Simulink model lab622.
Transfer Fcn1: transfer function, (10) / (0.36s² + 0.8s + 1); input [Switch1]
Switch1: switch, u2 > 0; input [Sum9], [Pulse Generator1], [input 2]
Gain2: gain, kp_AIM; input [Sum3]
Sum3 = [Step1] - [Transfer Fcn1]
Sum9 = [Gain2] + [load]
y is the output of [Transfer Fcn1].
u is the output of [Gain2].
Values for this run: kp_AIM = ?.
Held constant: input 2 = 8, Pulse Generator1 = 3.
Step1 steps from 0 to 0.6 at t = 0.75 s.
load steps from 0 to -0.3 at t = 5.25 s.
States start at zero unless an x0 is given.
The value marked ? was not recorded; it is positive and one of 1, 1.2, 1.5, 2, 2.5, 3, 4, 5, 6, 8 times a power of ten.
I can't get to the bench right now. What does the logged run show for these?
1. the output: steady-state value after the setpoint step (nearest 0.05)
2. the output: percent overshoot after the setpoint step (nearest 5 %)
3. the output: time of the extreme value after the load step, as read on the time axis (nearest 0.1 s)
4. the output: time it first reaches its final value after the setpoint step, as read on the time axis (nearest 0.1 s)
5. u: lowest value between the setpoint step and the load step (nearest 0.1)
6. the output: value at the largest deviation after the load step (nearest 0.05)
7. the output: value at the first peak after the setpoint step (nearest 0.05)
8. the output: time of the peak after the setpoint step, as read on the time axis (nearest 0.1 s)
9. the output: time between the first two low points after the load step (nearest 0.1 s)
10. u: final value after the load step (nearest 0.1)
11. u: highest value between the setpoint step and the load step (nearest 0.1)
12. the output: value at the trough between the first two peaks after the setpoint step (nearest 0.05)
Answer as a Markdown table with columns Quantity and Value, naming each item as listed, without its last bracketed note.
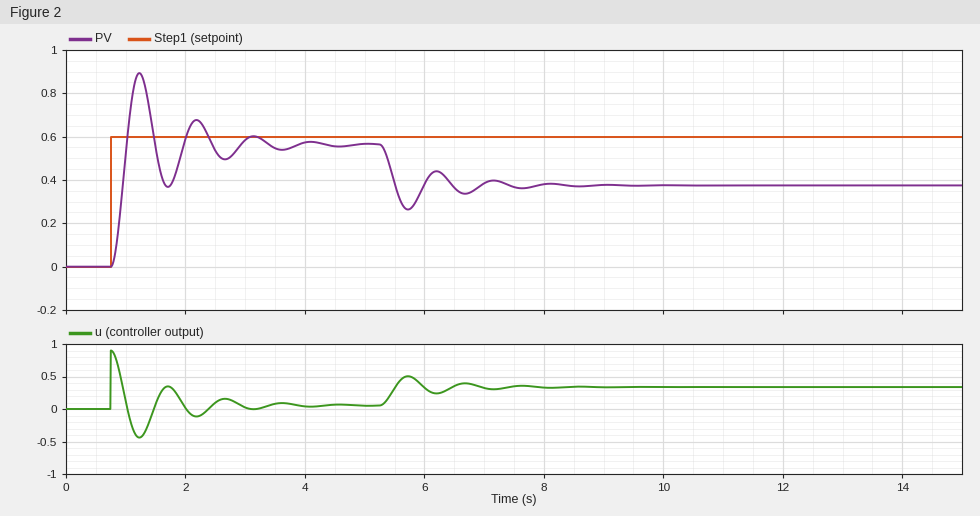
| Quantity | Value |
|---|---|
| the output: steady-state value after the setpoint step | 0.55 |
| the output: percent overshoot after the setpoint step | 60 % |
| the output: time of the extreme value after the load step, as read on the time axis | 5.7 s |
| the output: time it first reaches its final value after the setpoint step, as read on the time axis | 1.0 s |
| u: lowest value between the setpoint step and the load step | -0.4 |
| the output: value at the largest deviation after the load step | 0.25 |
| the output: value at the first peak after the setpoint step | 0.90 |
| the output: time of the peak after the setpoint step, as read on the time axis | 1.2 s |
| the output: time between the first two low points after the load step | 1.0 s |
| u: final value after the load step | 0.3 |
| u: highest value between the setpoint step and the load step | 0.9 |
| the output: value at the trough between the first two peaks after the setpoint step | 0.35 |
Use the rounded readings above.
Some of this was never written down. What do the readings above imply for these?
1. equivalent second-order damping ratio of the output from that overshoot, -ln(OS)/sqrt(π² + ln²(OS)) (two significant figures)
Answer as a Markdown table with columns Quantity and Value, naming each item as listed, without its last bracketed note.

| Quantity | Value |
|---|---|
| equivalent second-order damping ratio of the output from that overshoot, -ln(OS)/sqrt(π² + ln²(OS)) | 0.16 |
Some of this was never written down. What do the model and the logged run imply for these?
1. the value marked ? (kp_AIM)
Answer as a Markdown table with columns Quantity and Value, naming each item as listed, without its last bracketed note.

| Quantity | Value |
|---|---|
| the value marked ? | 1.5 |
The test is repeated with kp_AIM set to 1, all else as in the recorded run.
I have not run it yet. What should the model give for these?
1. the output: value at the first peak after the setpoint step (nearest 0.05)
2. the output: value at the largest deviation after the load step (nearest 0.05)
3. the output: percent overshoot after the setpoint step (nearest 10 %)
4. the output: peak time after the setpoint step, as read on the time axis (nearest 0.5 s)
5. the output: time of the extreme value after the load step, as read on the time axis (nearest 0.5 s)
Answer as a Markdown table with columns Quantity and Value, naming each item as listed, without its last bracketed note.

| Quantity | Value |
|---|---|
| the output: value at the first peak after the setpoint step | 0.85 |
| the output: value at the largest deviation after the load step | 0.15 |
| the output: percent overshoot after the setpoint step | 50 % |
| the output: peak time after the setpoint step, as read on the time axis | 1.5 s |
| the output: time of the extreme value after the load step, as read on the time axis | 6.0 s |
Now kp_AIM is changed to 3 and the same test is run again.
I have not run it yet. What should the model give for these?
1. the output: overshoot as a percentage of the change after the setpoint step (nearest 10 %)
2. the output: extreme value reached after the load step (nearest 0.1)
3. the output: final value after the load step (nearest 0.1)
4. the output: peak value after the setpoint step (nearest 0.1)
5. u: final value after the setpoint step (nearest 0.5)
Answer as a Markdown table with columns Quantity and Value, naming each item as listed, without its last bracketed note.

| Quantity | Value |
|---|---|
| the output: overshoot as a percentage of the change after the setpoint step | 70 % |
| the output: extreme value reached after the load step | 0.4 |
| the output: final value after the load step | 0.5 |
| the output: peak value after the setpoint step | 1.0 |
| u: final value after the setpoint step | 0.0 |
